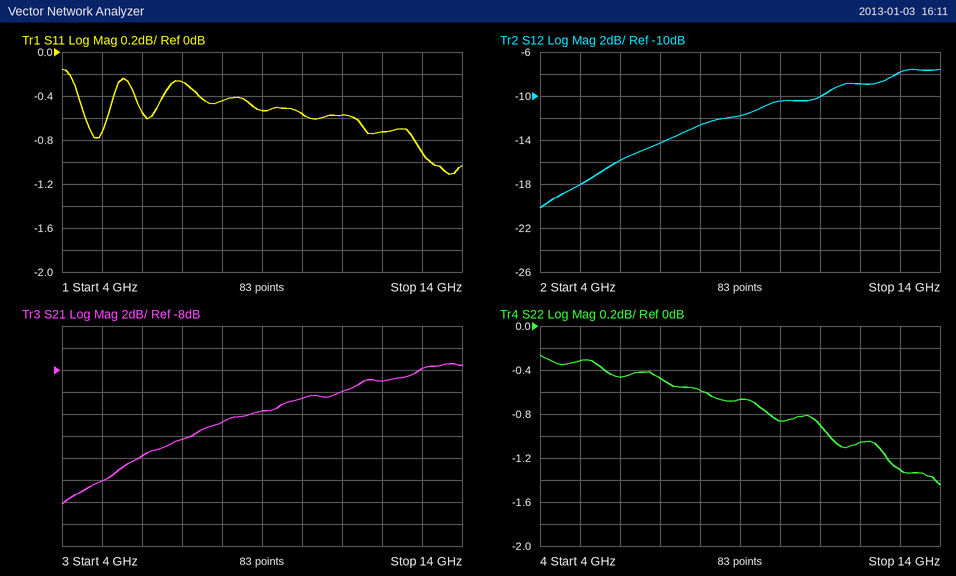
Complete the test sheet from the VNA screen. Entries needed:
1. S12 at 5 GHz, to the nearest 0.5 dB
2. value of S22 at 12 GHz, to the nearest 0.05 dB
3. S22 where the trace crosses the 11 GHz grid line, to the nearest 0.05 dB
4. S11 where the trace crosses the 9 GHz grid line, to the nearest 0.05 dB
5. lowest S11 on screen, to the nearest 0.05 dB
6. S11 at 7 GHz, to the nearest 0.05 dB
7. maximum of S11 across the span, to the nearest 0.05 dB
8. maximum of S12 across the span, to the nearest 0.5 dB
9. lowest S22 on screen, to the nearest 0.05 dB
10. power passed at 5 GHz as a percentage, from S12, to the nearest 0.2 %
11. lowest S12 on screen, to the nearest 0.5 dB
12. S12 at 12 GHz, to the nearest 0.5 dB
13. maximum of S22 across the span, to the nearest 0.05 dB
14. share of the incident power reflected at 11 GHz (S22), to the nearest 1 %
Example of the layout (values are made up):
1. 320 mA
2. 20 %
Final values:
1. -18.0 dB
2. -1.05 dB
3. -0.90 dB
4. -0.55 dB
5. -1.10 dB
6. -0.25 dB
7. -0.15 dB
8. -7.5 dB
9. -1.45 dB
10. 1.6 %
11. -20.0 dB
12. -9.0 dB
13. -0.25 dB
14. 81 %
